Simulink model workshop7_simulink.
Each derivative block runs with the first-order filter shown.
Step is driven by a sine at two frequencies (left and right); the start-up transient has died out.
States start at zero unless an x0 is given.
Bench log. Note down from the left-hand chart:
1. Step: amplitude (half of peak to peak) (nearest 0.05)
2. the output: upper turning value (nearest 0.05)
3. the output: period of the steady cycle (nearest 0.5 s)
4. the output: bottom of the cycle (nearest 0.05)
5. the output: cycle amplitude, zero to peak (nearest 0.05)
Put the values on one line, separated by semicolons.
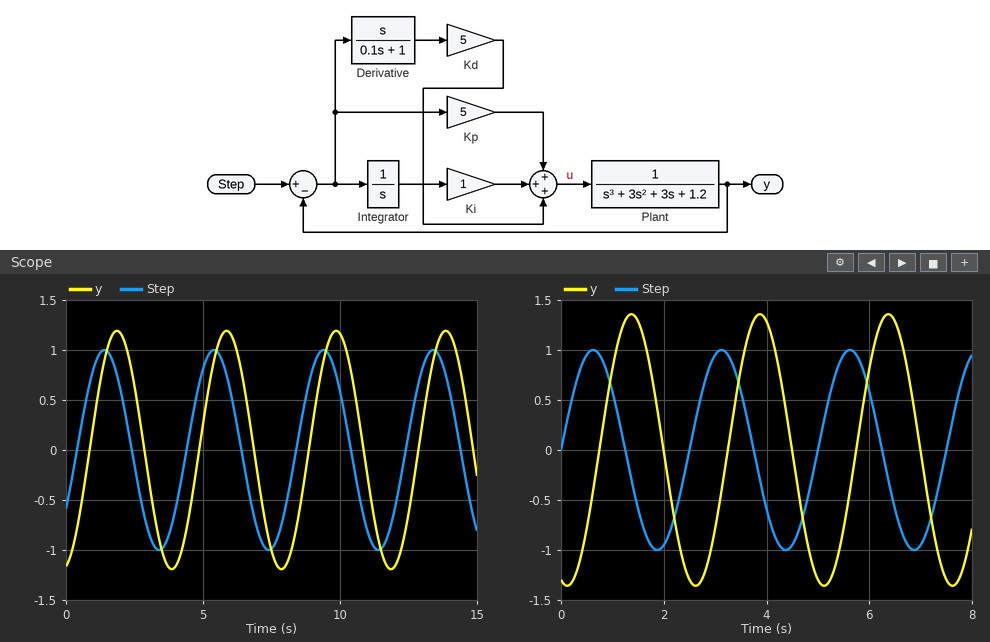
1.00; 1.20; 4.0 s; -1.20; 1.20
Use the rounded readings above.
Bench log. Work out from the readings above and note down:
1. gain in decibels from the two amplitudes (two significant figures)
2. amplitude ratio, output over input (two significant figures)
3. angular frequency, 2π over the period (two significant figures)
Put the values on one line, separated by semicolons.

1.6 dB; 1.2; 1.6 rad/s
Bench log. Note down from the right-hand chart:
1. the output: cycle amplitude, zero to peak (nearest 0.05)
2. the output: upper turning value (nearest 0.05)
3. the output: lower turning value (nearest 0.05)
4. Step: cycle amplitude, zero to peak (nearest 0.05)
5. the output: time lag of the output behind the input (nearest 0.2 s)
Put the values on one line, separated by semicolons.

1.35; 1.35; -1.35; 1.00; 0.8 s
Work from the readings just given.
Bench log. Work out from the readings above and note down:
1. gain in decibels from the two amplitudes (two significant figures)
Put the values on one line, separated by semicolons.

2.6 dB
